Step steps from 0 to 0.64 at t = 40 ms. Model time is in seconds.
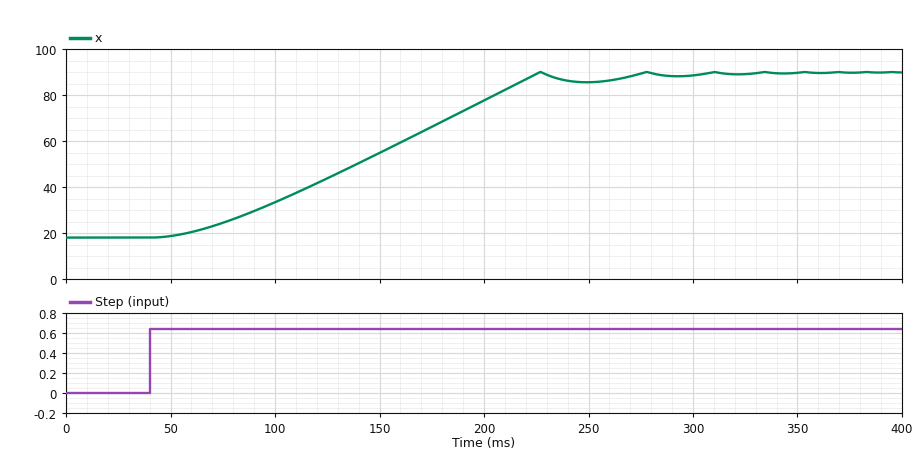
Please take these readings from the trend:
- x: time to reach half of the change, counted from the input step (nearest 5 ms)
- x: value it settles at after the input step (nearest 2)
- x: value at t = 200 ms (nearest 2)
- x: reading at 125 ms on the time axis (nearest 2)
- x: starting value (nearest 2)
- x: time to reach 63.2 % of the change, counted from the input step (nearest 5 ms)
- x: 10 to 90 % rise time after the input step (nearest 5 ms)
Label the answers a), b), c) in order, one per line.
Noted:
a) 110 ms
b) 90
c) 78
d) 44
e) 18
f) 130 ms
g) 135 ms
